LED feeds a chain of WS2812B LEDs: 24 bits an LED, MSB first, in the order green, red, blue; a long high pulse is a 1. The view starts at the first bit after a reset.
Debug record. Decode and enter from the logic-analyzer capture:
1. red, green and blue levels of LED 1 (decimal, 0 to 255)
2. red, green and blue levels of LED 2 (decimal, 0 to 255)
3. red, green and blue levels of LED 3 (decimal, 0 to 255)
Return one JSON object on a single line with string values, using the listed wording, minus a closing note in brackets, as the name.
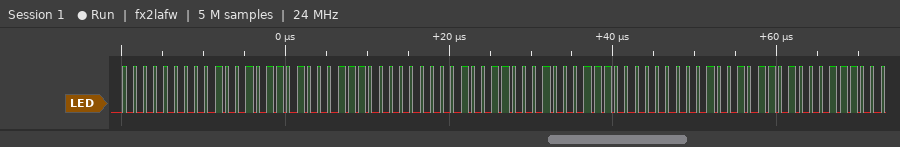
{"red, green and blue levels of LED 1": "75, 0, 71", "red, green and blue levels of LED 2": "76, 0, 71", "red, green and blue levels of LED 3": "75, 0, 71"}
